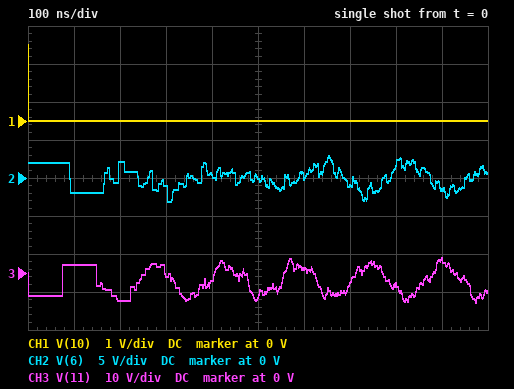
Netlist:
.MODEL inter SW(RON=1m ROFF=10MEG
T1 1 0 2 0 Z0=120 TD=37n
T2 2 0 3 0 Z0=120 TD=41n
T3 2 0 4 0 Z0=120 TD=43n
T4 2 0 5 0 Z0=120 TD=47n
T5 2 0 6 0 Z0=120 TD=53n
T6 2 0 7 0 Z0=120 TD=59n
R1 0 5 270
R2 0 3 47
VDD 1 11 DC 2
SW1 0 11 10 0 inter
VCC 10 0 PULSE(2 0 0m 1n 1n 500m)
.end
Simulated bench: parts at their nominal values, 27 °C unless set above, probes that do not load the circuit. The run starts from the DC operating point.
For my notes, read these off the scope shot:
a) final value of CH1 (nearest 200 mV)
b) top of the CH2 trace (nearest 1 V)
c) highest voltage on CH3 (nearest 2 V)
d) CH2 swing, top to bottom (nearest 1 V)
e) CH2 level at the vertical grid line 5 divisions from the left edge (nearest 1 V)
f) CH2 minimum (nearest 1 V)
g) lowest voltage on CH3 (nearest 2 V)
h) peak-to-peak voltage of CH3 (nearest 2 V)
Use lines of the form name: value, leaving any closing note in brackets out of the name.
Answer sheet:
final value of CH1: 0 V
top of the CH2 trace: 3 V
highest voltage on CH3: 4 V
CH2 swing, top to bottom: 6 V
CH2 level at the vertical grid line 5 divisions from the left edge: 0 V
CH2 minimum: -3 V
lowest voltage on CH3: -8 V
peak-to-peak voltage of CH3: 12 V
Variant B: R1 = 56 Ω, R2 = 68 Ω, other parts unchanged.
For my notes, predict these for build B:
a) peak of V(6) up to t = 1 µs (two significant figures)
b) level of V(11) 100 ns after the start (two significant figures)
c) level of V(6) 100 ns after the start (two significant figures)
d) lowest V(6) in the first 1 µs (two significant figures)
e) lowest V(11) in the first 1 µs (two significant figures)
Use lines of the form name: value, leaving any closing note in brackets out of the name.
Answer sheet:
peak of V(6) up to t = 1 µs: 3.7 V
level of V(11) 100 ns after the start: 2.6 V
level of V(6) 100 ns after the start: -3.2 V
lowest V(6) in the first 1 µs: -3.7 V
lowest V(11) in the first 1 µs: -9.5 V
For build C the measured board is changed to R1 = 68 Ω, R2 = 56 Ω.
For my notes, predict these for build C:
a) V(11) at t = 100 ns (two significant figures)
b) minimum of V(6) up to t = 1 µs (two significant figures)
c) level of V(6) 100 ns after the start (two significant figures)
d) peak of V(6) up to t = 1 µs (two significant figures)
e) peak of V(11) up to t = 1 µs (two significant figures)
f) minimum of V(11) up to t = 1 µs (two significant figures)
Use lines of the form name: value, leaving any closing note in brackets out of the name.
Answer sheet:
V(11) at t = 100 ns: 2.6 V
minimum of V(6) up to t = 1 µs: -3.8 V
level of V(6) 100 ns after the start: -3.2 V
peak of V(6) up to t = 1 µs: 3.7 V
peak of V(11) up to t = 1 µs: 5.6 V
minimum of V(11) up to t = 1 µs: -9.4 V
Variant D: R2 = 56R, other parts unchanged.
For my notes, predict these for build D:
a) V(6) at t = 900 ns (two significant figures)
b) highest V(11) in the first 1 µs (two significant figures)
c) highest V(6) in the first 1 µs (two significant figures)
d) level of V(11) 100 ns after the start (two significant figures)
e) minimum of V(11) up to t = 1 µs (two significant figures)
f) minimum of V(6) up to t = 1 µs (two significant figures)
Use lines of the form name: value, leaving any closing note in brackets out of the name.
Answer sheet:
V(6) at t = 900 ns: -1.2 V
highest V(11) in the first 1 µs: 3.1 V
highest V(6) in the first 1 µs: 2.4 V
level of V(11) 100 ns after the start: 1.7 V
minimum of V(11) up to t = 1 µs: -7.0 V
minimum of V(6) up to t = 1 µs: -2.7 V
